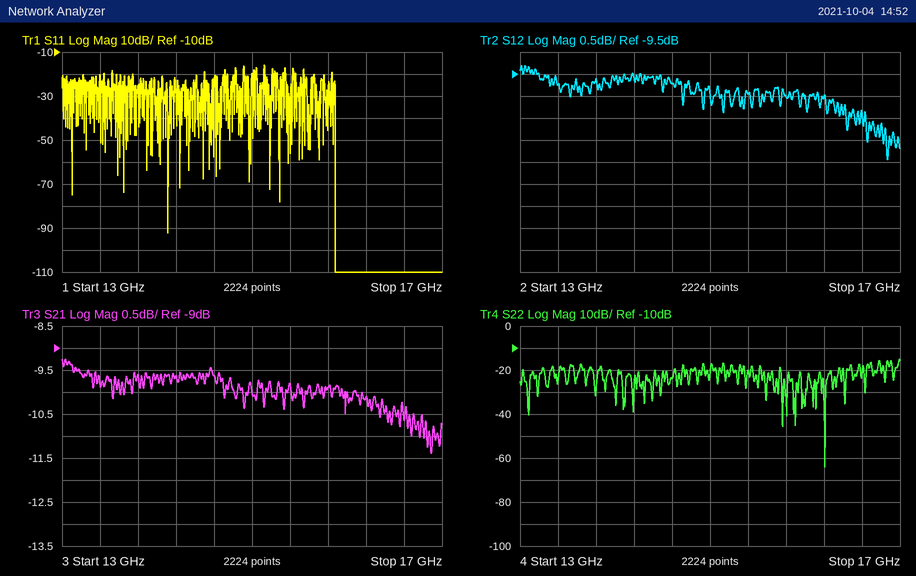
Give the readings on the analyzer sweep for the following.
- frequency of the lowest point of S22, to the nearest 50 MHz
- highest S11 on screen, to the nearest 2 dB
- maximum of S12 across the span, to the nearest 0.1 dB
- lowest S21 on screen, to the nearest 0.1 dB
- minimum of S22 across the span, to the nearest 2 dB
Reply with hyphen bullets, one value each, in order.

- 16.20 GHz
- -16 dB
- -9.3 dB
- -11.4 dB
- -64 dB
